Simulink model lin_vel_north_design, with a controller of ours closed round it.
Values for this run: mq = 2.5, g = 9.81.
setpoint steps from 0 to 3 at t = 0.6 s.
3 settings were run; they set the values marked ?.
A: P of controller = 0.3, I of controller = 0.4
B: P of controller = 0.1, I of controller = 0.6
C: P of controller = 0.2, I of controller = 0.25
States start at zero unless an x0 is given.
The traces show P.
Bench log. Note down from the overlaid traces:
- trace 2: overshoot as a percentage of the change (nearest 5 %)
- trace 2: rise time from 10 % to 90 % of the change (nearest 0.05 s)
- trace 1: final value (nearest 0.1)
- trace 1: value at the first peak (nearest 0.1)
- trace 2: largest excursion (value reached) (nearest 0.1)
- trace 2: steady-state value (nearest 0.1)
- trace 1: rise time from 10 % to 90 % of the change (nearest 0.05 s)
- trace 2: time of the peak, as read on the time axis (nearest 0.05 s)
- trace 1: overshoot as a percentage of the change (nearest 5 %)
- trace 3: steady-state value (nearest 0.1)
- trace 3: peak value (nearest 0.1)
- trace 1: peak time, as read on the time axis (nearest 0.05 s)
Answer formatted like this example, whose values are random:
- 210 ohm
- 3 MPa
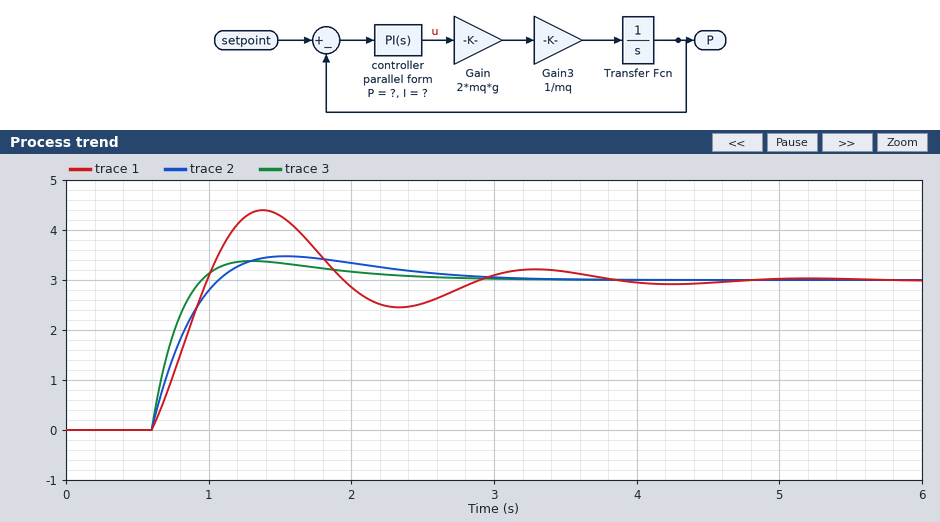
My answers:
- 15 %
- 0.35 s
- 3.0
- 4.4
- 3.5
- 3.0
- 0.30 s
- 1.55 s
- 45 %
- 3.0
- 3.4
- 1.40 s
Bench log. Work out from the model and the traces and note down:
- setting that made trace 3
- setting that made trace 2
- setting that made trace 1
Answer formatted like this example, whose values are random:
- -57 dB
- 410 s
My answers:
- A
- C
- B
